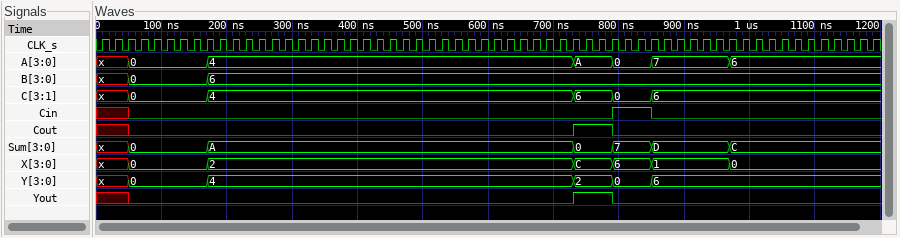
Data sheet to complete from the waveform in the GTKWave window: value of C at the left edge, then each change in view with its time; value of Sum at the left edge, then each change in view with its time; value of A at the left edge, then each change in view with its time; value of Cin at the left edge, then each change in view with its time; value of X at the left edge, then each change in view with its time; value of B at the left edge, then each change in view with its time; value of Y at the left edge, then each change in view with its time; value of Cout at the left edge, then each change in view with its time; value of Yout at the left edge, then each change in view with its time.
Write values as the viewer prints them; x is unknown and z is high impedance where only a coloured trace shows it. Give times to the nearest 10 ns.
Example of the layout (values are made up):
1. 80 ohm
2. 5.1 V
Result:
1. x, 0 at 50 ns, 4 at 170 ns, 6 at 730 ns, 0 at 790 ns, 6 at 850 ns
2. x, 0 at 50 ns, A at 170 ns, 0 at 730 ns, 7 at 790 ns, D at 850 ns, C at 970 ns
3. x, 0 at 50 ns, 4 at 170 ns, A at 730 ns, 0 at 790 ns, 7 at 850 ns, 6 at 970 ns
4. x, 0 at 50 ns, 1 at 790 ns, 0 at 850 ns
5. x, 0 at 50 ns, 2 at 170 ns, C at 730 ns, 6 at 790 ns, 1 at 850 ns, 0 at 970 ns
6. x, 0 at 50 ns, 6 at 170 ns
7. x, 0 at 50 ns, 4 at 170 ns, 2 at 730 ns, 0 at 790 ns, 6 at 850 ns
8. x, 0 at 50 ns, 1 at 730 ns, 0 at 790 ns
9. x, 0 at 50 ns, 1 at 730 ns, 0 at 790 ns
